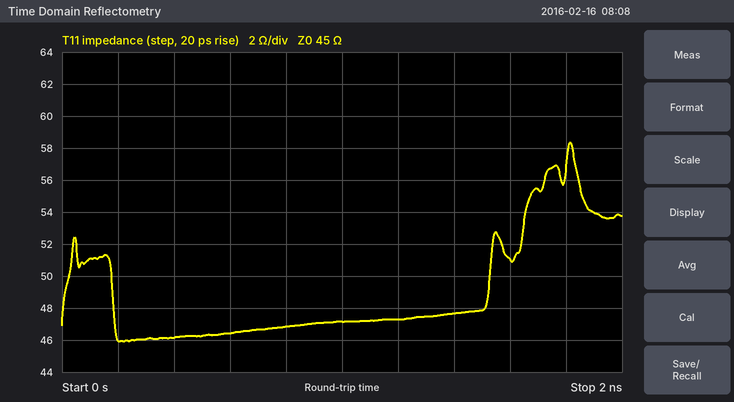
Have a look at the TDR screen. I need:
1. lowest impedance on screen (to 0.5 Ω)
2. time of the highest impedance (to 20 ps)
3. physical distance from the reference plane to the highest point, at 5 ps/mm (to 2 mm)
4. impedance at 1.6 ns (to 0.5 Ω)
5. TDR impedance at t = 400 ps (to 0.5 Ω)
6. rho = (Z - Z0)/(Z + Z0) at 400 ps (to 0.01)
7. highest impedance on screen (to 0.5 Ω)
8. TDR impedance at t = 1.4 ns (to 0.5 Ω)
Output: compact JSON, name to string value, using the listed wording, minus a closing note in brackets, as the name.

{"lowest impedance on screen": "46.0 Ω", "time of the highest impedance": "1.82 ns", "physical distance from the reference plane to the highest point, at 5 ps/mm": "182 mm", "impedance at 1.6 ns": "51.0 Ω", "TDR impedance at t = 400 ps": "46.0 Ω", "rho = (Z - Z0)/(Z + Z0) at 400 ps": "+0.01", "highest impedance on screen": "58.5 Ω", "TDR impedance at t = 1.4 ns": "47.5 Ω"}
